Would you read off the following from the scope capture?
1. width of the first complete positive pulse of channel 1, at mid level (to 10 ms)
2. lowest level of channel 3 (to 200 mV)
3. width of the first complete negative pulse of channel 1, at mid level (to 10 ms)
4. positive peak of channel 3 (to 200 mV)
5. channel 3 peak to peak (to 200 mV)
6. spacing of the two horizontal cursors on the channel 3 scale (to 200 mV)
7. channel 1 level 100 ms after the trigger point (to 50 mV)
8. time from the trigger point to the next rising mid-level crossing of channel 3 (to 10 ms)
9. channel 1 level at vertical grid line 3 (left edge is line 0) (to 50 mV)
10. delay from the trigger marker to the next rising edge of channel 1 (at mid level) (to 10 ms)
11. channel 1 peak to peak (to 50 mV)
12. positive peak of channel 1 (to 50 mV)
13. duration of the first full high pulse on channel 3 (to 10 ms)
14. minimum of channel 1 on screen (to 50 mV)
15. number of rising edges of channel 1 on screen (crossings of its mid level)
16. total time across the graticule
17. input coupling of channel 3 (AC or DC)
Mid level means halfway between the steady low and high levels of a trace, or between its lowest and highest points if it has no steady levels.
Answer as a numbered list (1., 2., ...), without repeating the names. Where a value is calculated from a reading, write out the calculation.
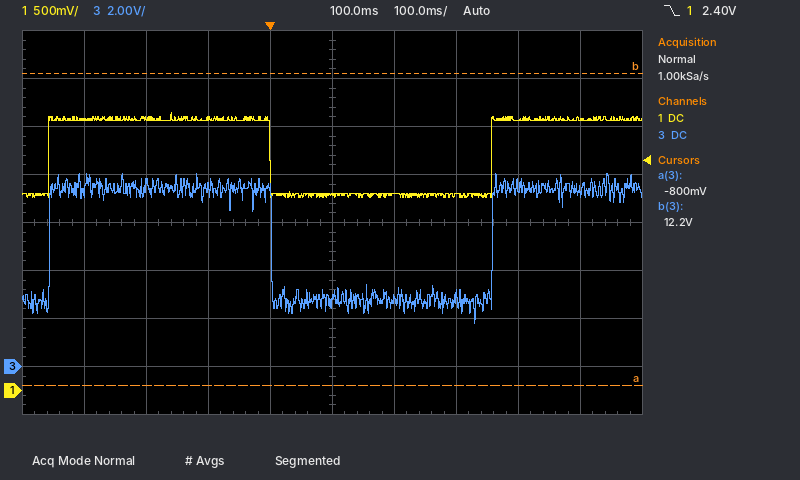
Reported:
1. 360 ms
2. 1.8 V
3. 360 ms
4. 8.0 V
5. 8.0 V − (1.8 V) = 6.2 V
6. 13.0 V
7. 2.05 V
8. 360 ms
9. 2.85 V
10. 360 ms
11. 2.90 V − (2.00 V) = 900 mV
12. 2.90 V
13. 360 ms
14. 2.00 V
15. 2
16. 1 s
17. DC
